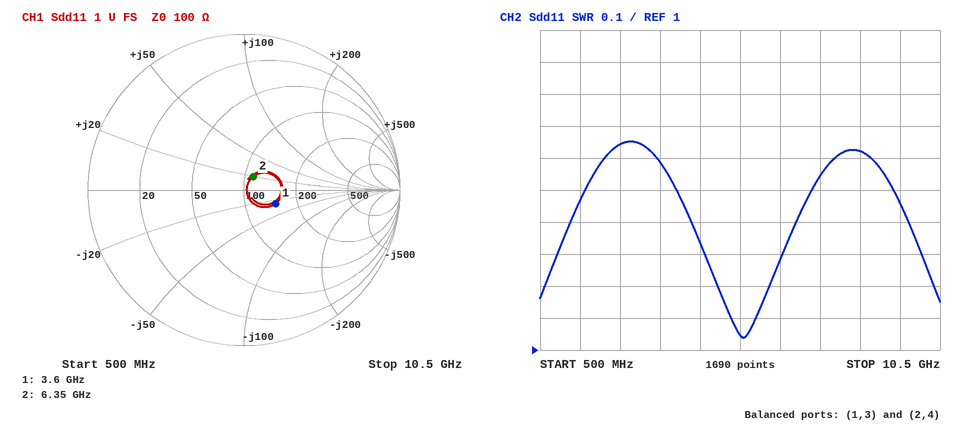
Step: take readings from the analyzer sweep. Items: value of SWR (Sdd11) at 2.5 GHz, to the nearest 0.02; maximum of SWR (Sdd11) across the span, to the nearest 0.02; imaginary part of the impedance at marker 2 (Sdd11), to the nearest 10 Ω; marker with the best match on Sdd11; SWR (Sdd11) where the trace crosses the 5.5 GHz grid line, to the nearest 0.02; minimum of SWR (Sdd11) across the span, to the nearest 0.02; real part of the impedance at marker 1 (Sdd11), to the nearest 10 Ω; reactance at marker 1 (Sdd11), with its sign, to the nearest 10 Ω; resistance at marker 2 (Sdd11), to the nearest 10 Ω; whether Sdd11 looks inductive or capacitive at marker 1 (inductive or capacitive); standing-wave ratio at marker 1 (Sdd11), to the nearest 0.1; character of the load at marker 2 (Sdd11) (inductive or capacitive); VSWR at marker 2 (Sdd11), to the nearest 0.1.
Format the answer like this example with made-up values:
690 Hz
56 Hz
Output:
1.64
1.66
+20 Ω
marker 2
1.04
1.04
150 Ω
-30 Ω
110 Ω
capacitive
1.6
inductive
1.2
